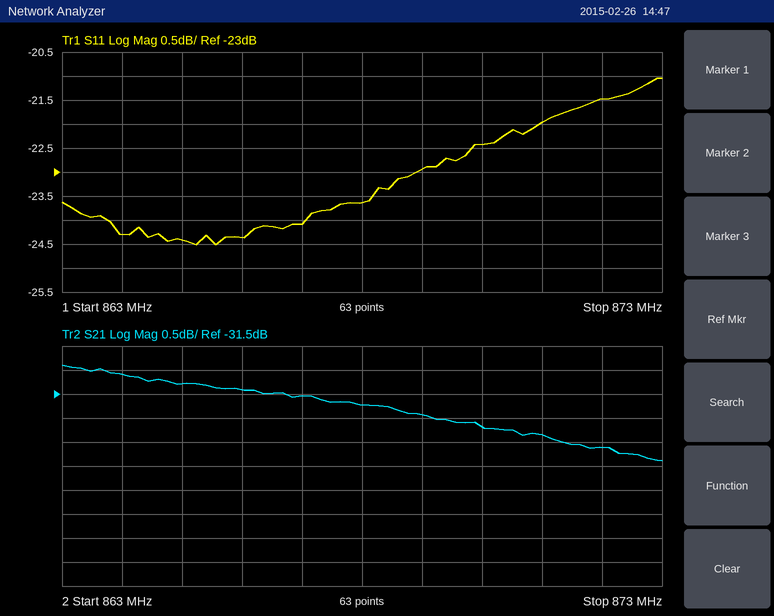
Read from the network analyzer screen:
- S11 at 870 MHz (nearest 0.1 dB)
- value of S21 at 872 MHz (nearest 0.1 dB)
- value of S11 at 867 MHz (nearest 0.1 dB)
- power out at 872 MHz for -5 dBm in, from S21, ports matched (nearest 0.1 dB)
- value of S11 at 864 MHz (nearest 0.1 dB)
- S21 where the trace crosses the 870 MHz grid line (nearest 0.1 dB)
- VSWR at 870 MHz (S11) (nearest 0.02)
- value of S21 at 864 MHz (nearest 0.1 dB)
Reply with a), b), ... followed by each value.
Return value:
a) -22.4 dB
b) -32.6 dB
c) -24.1 dB
d) -37.6 dBm
e) -24.3 dB
f) -32.2 dB
g) 1.16
h) -31.1 dB
